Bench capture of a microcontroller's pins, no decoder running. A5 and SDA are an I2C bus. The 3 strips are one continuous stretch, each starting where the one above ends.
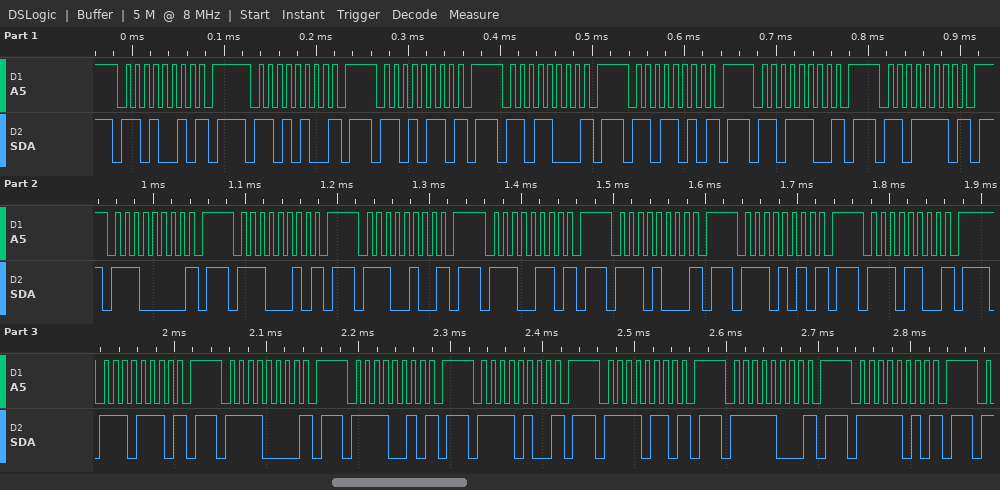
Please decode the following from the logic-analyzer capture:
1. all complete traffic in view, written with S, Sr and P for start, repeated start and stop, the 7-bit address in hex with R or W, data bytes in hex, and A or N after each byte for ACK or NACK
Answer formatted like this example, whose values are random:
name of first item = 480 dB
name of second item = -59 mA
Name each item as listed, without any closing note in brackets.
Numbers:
all complete traffic in view, written with S, Sr and P for start, repeated start and stop, the 7-bit address in hex with R or W, data bytes in hex, and A or N after each byte for ACK or NACK = S 69W N P S 6AW N P S 6BW N P S 6CW N P S 6DW N P S 6EW N P S 6FW N P S 70W N P S 71W N P S 72W N P S 73W N P S 74W N P S 75W N P S 76W N P S 77W N P S 78W N P S 79W N P S 7AW N P S 7BW N P S 7CW N P S 7DW N P
